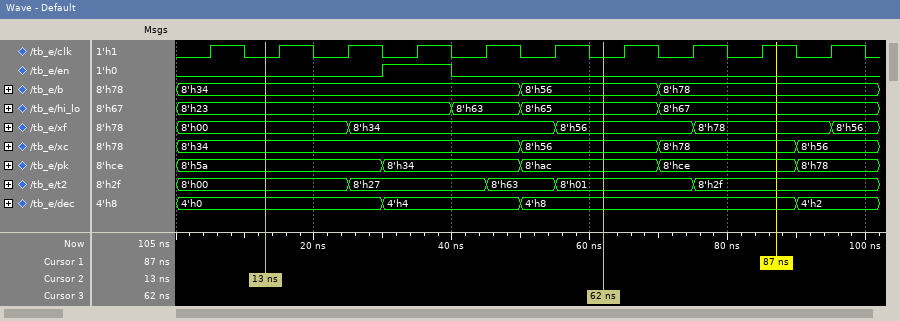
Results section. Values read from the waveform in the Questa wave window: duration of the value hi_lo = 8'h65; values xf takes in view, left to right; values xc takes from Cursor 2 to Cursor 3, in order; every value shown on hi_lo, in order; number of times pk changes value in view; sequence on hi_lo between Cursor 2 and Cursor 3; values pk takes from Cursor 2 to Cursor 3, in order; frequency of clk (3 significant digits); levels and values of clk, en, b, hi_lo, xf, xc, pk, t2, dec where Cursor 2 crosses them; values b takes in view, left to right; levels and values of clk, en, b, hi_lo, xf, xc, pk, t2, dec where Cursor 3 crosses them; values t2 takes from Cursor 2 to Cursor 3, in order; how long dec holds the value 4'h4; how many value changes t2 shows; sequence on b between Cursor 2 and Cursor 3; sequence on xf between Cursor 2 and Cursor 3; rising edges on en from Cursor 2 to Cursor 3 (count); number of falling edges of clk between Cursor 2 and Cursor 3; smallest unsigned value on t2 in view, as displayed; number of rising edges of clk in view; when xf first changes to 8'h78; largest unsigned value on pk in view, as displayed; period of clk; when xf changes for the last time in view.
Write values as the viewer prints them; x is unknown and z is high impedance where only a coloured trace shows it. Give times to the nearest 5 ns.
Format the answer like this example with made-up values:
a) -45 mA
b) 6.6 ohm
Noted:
a) 20 ns
b) 8'h00, 8'h34, 8'h56, 8'h78, 8'h56
c) 8'h34, 8'h56
d) 8'h23, 8'h63, 8'h65, 8'h67
e) 4
f) 8'h23, 8'h63, 8'h65
g) 8'h5a, 8'h34, 8'hac
h) 100 MHz
i) clk=0, en=0, b=8'h34, hi_lo=8'h23, xf=8'h00, xc=8'h34, pk=8'h5a, t2=8'h00, dec=4'h0
j) 8'h34, 8'h56, 8'h78
k) clk=0, en=0, b=8'h56, hi_lo=8'h65, xf=8'h56, xc=8'h56, pk=8'hac, t2=8'h01, dec=4'h8
l) 8'h00, 8'h27, 8'h63, 8'h01
m) 20 ns
n) 4
o) 8'h34, 8'h56
p) 8'h00, 8'h34, 8'h56
q) 1
r) 5
s) 8'h00
t) 10
u) 75 ns
v) 8'hce
w) 10 ns
x) 95 ns
